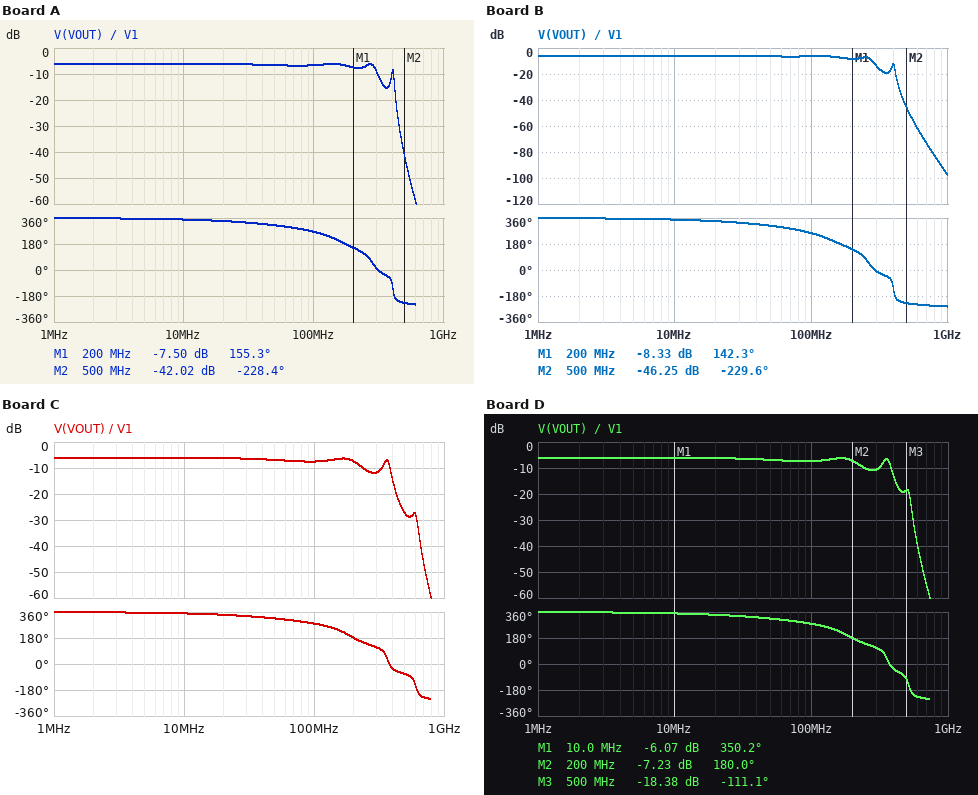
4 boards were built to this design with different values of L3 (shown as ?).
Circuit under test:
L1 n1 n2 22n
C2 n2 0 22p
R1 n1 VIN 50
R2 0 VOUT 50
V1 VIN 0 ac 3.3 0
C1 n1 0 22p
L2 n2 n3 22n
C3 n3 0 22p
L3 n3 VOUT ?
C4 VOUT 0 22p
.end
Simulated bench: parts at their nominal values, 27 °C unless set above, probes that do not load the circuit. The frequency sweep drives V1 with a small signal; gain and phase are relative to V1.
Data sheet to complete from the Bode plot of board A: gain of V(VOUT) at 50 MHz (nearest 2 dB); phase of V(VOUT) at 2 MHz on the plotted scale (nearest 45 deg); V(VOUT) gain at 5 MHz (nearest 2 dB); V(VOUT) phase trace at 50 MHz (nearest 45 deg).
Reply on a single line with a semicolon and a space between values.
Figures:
-6 dB; 360 deg; -6 dB; 315 deg
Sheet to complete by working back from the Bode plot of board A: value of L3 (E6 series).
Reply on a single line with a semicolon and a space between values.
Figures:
33 nH
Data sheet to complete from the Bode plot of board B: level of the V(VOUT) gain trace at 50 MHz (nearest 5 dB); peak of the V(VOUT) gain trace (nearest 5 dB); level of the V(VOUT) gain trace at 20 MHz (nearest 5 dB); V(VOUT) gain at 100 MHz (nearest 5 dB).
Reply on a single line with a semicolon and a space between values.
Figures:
-5 dB; -5 dB; -5 dB; -5 dB
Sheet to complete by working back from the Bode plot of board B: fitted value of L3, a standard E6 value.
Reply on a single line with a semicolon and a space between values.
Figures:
47 nH
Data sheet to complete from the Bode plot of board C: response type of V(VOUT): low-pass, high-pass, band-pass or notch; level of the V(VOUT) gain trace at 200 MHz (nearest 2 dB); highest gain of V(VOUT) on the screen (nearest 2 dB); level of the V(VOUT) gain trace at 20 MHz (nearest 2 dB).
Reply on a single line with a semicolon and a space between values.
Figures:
low-pass; -8 dB; -6 dB; -6 dB
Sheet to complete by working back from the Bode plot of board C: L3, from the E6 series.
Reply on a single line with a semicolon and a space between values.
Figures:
6.8 nH
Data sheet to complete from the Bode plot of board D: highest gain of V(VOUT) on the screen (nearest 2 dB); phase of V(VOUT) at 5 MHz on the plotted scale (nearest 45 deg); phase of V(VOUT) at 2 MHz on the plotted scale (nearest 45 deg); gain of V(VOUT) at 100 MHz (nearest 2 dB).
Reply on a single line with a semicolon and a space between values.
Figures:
-6 dB; 360 deg; 360 deg; -8 dB
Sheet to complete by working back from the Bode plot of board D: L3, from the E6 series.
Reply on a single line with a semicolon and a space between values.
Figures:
10 nH
